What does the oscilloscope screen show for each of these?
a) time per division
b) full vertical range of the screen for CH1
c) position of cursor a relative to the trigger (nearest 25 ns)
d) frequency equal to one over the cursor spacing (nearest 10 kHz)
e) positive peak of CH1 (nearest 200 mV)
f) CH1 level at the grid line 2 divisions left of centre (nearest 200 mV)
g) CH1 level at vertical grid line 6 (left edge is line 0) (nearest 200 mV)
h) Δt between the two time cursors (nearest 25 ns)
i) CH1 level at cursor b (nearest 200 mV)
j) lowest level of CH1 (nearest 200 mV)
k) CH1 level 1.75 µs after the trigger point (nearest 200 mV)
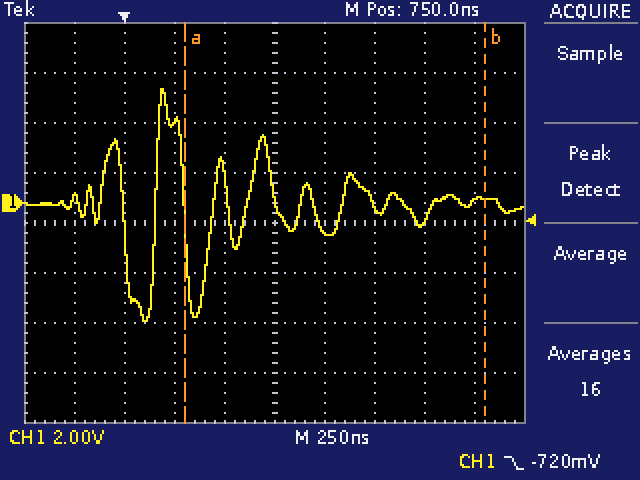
250 ns
16 V
+300 ns
670 kHz
4.6 V
3.2 V
-1.2 V
1.500 µs
200 mV
-4.8 V
0.0 V
